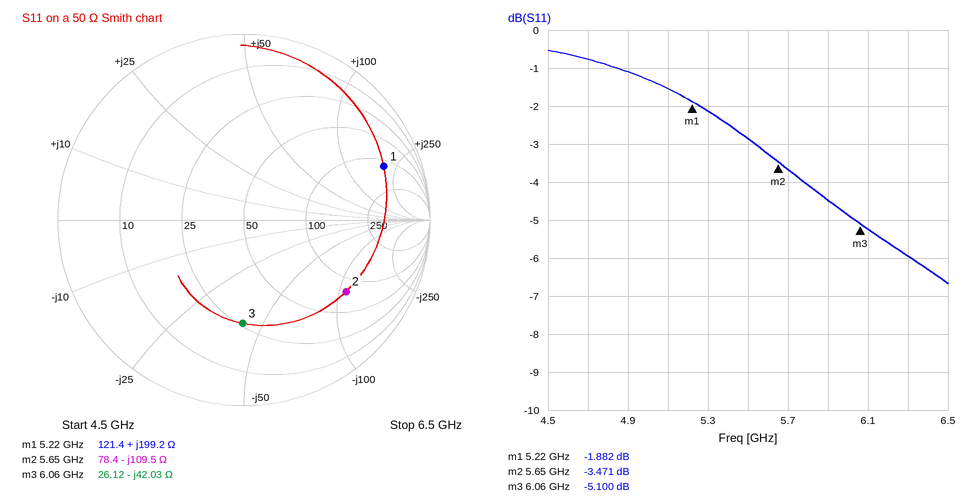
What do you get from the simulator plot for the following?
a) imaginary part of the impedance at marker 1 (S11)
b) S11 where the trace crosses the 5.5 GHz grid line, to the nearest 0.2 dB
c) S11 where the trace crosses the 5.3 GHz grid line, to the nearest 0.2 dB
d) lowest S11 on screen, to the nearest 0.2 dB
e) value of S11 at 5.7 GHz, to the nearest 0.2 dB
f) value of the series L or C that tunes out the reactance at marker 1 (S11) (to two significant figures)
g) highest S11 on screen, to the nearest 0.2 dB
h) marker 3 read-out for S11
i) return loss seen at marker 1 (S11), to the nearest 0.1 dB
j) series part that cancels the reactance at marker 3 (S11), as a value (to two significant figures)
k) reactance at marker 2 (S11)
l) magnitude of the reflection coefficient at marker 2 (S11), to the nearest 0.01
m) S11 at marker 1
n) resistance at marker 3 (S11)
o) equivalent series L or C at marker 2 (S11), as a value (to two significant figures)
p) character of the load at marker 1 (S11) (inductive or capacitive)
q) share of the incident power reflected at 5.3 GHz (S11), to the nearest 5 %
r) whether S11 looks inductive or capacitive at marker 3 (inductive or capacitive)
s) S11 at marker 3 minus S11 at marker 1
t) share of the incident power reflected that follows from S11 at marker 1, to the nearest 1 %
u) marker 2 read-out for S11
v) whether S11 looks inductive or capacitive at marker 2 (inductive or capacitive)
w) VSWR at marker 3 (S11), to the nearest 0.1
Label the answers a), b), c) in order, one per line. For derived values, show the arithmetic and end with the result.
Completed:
a) +199.2 Ω
b) -2.8 dB
c) -2.2 dB
d) -6.6 dB
e) -3.6 dB
f) C = 1/(2π × 5.22 GHz × 199.2 Ω) ≈ 153 fF, so 150 fF to two significant figures
g) -0.6 dB
h) -5.100 dB
i) 1.9 dB
j) L = 42.03 Ω/(2π × 6.06 GHz) ≈ 1.1 nH
k) -109.5 Ω
l) 0.67
m) -1.882 dB
n) 26.12 Ω
o) C = 1/(2π × 5.65 GHz × 109.5 Ω) ≈ 257 fF, so 260 fF to two significant figures
p) inductive
q) 10^(-2.2/10) ≈ 60 %
r) capacitive
s) -5.1 − (-1.882) = -3.218 dB
t) 10^(-1.882/10) ≈ 65 %
u) -3.471 dB
v) capacitive
w) (1 + 0.5559)/(1 − 0.5559) ≈ 3.5
